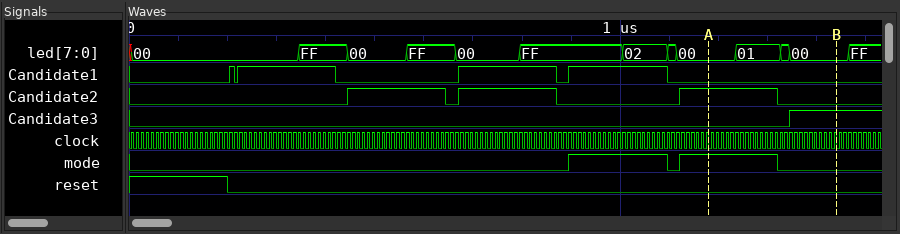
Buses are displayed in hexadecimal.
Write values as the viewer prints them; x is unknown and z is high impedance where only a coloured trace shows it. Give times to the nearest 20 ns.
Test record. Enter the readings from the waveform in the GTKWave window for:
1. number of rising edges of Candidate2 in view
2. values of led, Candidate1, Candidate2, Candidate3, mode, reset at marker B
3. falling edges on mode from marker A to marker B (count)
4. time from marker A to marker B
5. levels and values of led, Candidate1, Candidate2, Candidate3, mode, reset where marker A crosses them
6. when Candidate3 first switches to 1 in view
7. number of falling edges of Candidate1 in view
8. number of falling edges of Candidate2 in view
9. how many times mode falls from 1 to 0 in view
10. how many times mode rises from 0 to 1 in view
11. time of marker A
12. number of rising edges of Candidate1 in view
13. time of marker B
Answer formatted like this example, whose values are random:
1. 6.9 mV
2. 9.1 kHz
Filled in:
1. 3
2. led=00, Candidate1=0, Candidate2=0, Candidate3=1, mode=0, reset=0
3. 1
4. 260 ns
5. led=00, Candidate1=0, Candidate2=1, Candidate3=0, mode=1, reset=0
6. 1340 ns
7. 4
8. 3
9. 2
10. 2
11. 1180 ns
12. 4
13. 1440 ns
